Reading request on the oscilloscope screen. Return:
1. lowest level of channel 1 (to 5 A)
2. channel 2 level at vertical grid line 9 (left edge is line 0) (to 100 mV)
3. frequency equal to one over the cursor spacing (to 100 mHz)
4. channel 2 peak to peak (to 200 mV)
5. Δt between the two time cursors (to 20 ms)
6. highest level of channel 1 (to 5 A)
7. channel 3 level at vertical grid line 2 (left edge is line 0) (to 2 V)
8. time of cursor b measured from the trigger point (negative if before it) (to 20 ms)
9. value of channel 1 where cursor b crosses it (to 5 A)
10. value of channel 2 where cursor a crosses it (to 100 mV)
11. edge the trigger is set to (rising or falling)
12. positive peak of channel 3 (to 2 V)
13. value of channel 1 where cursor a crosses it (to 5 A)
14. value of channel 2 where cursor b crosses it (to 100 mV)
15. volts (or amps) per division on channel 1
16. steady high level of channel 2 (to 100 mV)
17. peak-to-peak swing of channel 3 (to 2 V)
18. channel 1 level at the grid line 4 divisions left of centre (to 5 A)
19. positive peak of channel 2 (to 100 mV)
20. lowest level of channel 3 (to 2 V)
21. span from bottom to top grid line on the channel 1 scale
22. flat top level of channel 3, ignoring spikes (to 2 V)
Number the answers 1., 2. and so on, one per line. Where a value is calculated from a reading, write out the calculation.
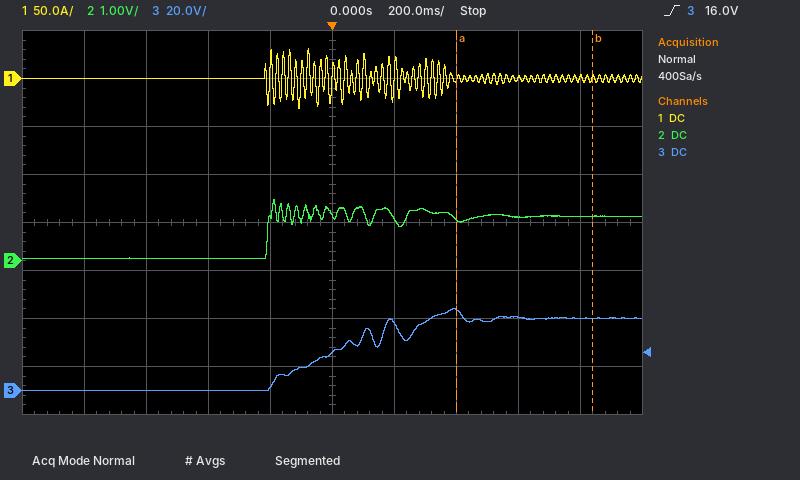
1. -30 A
2. 900 mV
3. 1 / 440 ms ≈ 2.3 Hz
4. 1.2 V
5. 440 ms
6. 30 A
7. 0 V
8. +840 ms
9. 0 A
10. 900 mV
11. rising
12. 34 V
13. 0 A
14. 900 mV
15. 50 A
16. 900 mV
17. 34 V − (0 V) = 34 V
18. 0 A
19. 1.3 V
20. 0 V
21. 400 A
22. 30 V
